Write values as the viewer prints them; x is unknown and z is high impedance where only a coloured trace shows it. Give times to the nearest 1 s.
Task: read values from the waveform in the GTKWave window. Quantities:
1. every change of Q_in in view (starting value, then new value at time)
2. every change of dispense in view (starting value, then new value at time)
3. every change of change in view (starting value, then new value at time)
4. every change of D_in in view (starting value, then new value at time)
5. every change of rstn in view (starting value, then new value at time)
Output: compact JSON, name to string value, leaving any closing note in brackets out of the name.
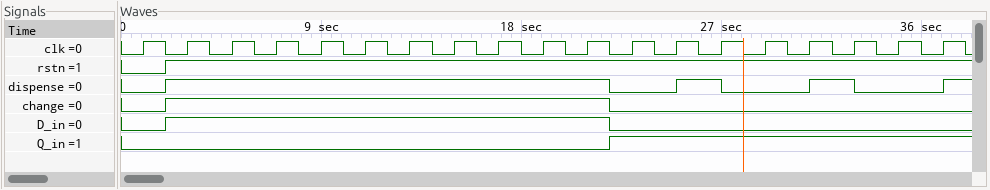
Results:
{"every change of Q_in in view": "0, 1 at 22 s", "every change of dispense in view": "0, 1 at 2 s, 0 at 22 s, 1 at 25 s, 0 at 27 s, 1 at 31 s, 0 at 33 s, 1 at 37 s", "every change of change in view": "0, 1 at 2 s, 0 at 22 s", "every change of D_in in view": "0, 1 at 2 s, 0 at 22 s", "every change of rstn in view": "0, 1 at 2 s"}
